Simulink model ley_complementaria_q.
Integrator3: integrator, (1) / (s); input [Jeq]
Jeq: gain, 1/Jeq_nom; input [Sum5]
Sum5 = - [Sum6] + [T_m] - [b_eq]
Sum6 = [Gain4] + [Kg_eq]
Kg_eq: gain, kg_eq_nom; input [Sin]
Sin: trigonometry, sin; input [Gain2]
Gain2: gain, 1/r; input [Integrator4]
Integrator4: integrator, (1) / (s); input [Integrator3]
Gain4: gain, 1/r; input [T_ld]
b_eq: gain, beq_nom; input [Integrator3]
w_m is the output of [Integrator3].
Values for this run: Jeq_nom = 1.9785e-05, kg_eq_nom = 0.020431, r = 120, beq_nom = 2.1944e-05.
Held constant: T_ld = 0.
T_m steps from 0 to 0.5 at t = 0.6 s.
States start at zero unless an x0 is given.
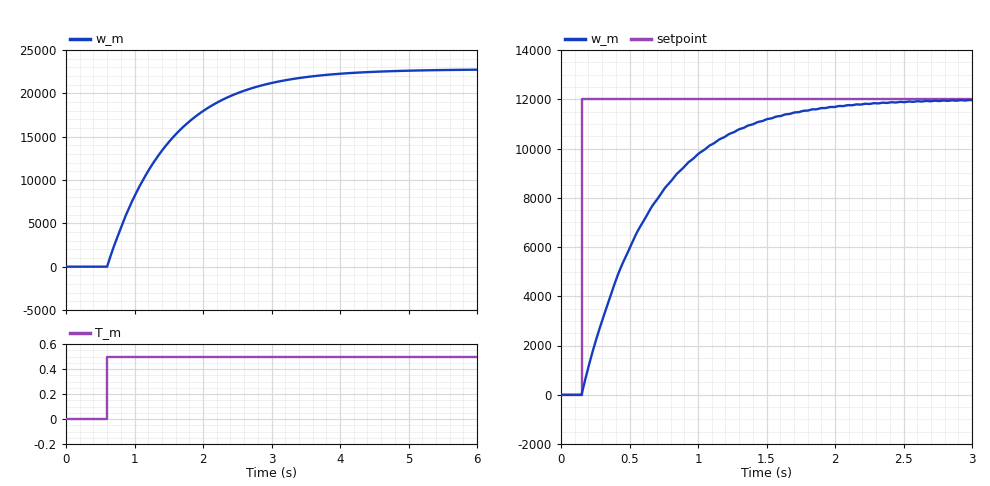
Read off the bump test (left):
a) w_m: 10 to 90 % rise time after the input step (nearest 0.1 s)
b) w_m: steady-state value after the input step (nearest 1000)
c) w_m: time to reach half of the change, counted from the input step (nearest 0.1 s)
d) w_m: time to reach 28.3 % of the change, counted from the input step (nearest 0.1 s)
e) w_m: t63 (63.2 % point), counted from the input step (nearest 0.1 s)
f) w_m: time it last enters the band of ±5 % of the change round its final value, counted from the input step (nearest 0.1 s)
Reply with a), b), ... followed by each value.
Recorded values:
a) 2.0 s
b) 23000
c) 0.6 s
d) 0.3 s
e) 0.9 s
f) 2.7 s
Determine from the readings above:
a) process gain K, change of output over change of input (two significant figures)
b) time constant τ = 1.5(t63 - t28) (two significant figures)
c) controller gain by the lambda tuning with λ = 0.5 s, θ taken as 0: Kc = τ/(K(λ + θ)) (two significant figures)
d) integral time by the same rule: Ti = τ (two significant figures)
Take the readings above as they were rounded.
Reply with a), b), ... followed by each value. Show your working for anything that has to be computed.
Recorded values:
a) (23000 - 0) / 0.5 = 46000
b) 1.5 × (0.9 - 0.3) = 0.90 s
c) 0.9 / (46000 × (0.5 + 0)) = 0.000039
d) 0.90 s
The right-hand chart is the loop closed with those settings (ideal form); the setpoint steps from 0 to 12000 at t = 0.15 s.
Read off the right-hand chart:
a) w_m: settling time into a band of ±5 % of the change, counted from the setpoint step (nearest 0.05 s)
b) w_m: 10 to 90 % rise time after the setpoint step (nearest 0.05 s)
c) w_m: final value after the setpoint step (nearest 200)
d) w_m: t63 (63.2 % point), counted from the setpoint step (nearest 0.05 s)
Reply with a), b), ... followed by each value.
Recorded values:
a) 1.50 s
b) 1.10 s
c) 12000
d) 0.50 s
